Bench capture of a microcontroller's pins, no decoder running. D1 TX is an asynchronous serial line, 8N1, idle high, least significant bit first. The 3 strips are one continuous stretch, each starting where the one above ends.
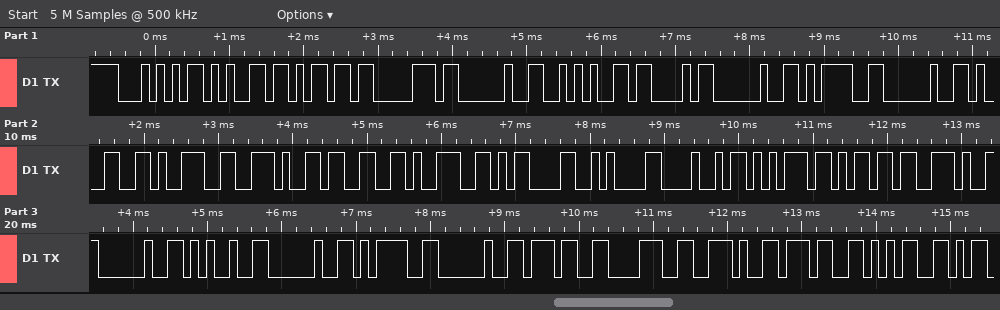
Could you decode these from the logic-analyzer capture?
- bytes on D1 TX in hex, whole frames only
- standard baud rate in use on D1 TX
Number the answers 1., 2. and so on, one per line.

1. 54 65 6D 70 20 2A 43 20 3D 20 31 39 2E 33 39 0D 0A 48 75 6D 2E 20 25 20 3D 20 37 38 2E 37 35
2. 9600 baud
